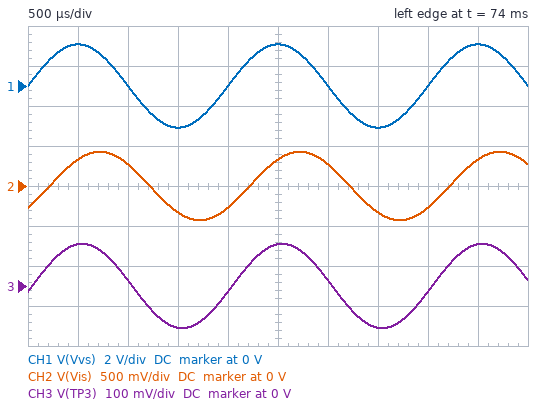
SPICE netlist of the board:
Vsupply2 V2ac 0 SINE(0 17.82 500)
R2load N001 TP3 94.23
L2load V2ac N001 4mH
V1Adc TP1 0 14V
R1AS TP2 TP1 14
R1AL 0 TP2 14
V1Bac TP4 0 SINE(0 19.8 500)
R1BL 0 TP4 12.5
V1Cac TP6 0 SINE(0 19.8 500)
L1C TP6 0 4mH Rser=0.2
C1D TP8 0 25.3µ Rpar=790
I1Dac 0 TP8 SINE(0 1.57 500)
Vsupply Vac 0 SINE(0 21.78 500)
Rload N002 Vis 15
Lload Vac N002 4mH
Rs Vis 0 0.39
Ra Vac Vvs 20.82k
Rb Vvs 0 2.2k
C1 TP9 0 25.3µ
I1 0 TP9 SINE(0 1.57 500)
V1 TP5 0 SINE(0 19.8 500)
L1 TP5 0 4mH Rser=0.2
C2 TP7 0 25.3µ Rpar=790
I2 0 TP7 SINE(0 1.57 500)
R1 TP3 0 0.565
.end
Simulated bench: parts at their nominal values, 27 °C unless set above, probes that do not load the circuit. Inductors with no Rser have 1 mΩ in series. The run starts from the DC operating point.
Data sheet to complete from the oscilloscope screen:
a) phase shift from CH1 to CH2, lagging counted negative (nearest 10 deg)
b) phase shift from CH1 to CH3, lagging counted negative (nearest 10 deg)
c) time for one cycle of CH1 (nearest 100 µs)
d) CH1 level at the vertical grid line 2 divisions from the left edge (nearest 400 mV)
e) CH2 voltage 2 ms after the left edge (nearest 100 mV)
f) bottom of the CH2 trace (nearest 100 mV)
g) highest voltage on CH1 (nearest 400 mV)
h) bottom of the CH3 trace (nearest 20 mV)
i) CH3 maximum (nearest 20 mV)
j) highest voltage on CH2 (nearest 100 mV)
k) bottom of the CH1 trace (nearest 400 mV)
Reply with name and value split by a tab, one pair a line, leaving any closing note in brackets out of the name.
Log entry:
phase shift from CH1 to CH2, lagging counted negative	-40 deg
phase shift from CH1 to CH3, lagging counted negative	-10 deg
time for one cycle of CH1	2.0 ms
CH1 level at the vertical grid line 2 divisions from the left edge	0 V
CH2 voltage 2 ms after the left edge	-300 mV
bottom of the CH2 trace	-400 mV
highest voltage on CH1	2.0 V
bottom of the CH3 trace	-100 mV
CH3 maximum	100 mV
highest voltage on CH2	400 mV
bottom of the CH1 trace	-2.0 V
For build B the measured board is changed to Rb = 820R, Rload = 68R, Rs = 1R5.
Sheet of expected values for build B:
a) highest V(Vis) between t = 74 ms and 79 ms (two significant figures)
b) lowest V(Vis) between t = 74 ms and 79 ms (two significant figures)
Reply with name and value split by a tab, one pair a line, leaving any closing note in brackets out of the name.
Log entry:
highest V(Vis) between t = 74 ms and 79 ms	460 mV
lowest V(Vis) between t = 74 ms and 79 ms	-460 mV
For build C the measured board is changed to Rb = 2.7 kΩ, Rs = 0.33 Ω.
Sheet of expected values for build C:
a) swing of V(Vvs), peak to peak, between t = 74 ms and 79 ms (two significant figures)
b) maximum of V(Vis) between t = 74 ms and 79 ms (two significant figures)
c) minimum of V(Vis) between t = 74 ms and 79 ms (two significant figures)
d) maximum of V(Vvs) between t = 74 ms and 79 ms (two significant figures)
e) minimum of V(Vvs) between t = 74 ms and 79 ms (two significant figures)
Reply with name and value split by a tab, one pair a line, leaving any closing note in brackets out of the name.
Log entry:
swing of V(Vvs), peak to peak, between t = 74 ms and 79 ms	5.0 V
maximum of V(Vis) between t = 74 ms and 79 ms	360 mV
minimum of V(Vis) between t = 74 ms and 79 ms	-360 mV
maximum of V(Vvs) between t = 74 ms and 79 ms	2.5 V
minimum of V(Vvs) between t = 74 ms and 79 ms	-2.5 V
